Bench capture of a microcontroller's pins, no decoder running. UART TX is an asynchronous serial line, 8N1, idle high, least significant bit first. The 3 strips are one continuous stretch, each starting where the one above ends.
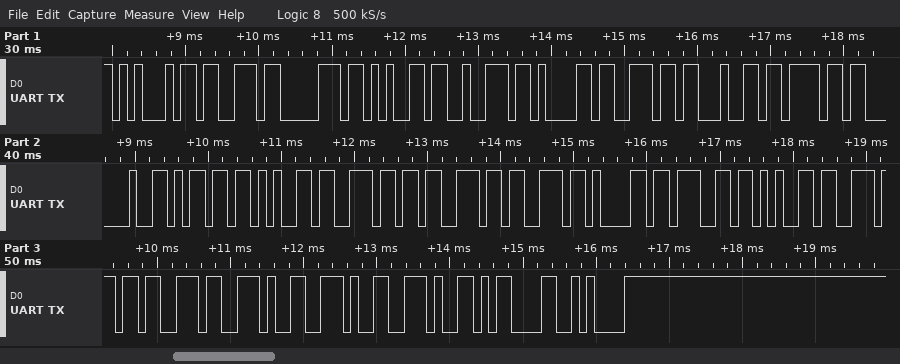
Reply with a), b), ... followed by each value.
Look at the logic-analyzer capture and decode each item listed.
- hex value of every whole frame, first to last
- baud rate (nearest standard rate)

a) 45 73 70 65 72 61 6E 64 6F 20 6D 65 6E 73 73 61 67 65 6E 73 2E 2E 2E 0D 0A
b) 9600 baud
